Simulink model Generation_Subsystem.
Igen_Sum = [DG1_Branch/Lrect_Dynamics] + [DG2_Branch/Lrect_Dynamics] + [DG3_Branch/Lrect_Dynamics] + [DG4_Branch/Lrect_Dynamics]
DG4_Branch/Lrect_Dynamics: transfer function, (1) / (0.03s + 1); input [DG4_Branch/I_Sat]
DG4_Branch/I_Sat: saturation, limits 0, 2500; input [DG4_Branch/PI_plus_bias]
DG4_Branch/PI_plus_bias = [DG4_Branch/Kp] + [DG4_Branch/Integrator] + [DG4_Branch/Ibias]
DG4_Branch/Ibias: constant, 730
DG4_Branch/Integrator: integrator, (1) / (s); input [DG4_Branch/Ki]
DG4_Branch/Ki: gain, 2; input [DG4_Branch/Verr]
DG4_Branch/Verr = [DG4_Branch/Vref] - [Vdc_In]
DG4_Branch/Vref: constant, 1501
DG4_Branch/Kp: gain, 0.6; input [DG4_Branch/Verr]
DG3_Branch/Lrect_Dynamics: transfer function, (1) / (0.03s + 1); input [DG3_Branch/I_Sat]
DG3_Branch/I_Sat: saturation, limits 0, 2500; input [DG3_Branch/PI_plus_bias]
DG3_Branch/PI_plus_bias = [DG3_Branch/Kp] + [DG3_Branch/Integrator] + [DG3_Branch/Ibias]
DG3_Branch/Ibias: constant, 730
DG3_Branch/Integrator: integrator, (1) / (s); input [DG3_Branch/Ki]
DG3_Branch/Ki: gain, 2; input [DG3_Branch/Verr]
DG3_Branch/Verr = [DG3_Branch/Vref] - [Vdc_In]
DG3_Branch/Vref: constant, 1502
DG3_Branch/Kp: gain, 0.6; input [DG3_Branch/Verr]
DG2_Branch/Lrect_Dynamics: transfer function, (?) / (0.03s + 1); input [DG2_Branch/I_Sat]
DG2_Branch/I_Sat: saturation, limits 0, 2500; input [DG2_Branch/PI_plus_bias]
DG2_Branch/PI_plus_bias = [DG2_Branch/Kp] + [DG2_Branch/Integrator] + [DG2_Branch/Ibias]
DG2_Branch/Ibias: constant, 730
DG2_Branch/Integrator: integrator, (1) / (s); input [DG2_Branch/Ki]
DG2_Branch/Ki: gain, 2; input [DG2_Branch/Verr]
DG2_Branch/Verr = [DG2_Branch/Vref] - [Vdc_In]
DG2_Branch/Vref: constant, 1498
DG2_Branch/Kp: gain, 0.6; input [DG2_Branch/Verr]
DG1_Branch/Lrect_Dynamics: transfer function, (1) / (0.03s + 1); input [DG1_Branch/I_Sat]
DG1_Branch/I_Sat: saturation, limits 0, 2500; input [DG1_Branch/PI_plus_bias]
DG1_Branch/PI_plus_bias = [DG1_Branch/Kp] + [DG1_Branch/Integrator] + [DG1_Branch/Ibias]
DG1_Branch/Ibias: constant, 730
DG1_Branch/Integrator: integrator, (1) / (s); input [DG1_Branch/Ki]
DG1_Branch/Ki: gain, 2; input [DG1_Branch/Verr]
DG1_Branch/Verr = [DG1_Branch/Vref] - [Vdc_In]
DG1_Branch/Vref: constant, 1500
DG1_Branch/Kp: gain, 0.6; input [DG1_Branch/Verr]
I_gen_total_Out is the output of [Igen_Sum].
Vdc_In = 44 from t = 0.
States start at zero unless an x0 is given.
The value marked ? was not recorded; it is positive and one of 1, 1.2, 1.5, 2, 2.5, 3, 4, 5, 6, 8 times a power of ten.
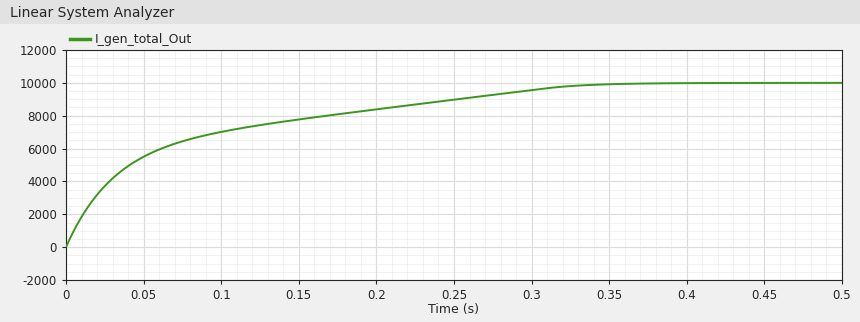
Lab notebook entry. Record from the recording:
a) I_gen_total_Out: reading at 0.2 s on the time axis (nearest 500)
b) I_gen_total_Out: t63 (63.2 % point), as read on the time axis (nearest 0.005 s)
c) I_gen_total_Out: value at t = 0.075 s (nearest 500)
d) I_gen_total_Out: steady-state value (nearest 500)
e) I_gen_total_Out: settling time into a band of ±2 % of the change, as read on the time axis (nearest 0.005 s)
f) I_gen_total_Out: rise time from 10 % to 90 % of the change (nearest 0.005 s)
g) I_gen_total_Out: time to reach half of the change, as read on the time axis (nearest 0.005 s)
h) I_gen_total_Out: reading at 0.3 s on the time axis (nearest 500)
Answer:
8500
0.070 s
6500
10000
0.325 s
0.245 s
0.040 s
9500
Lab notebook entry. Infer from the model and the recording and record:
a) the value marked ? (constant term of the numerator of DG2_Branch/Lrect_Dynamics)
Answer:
1
